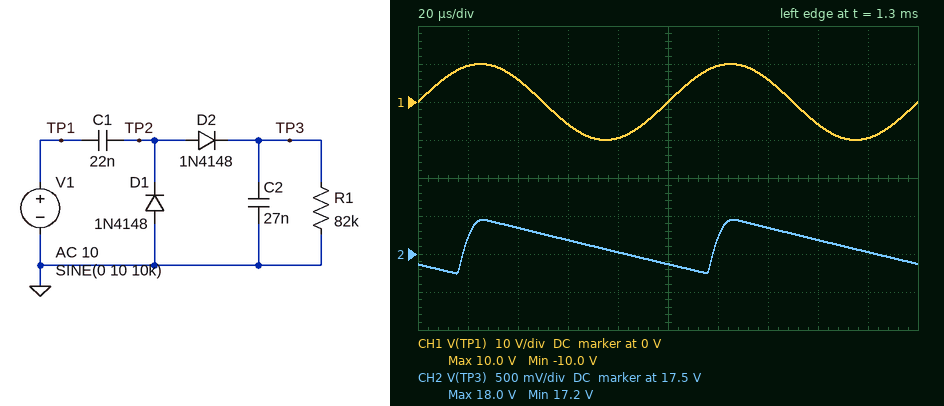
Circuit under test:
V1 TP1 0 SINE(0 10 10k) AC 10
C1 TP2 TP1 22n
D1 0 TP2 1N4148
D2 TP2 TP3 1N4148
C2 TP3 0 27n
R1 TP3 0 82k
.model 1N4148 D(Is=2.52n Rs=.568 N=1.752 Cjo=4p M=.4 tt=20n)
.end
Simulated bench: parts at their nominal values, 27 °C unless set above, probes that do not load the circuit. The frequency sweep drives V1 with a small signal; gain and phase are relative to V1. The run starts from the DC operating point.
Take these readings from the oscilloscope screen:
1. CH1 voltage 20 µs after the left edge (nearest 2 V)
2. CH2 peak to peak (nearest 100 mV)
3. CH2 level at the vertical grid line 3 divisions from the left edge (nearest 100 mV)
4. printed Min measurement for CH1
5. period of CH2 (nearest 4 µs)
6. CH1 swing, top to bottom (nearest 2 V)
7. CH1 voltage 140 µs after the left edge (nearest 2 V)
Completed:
10 V
700 mV
17.7 V
-10.0 V
100 µs
20 V
6 V
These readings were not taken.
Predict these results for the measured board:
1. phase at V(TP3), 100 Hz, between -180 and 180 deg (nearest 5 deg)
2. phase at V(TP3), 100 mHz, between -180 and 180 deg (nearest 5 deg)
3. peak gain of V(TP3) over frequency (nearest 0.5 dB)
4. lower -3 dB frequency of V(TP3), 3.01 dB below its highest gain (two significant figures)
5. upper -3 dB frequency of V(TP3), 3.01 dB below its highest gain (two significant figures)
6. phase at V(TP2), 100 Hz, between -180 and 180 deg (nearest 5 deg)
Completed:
-50 deg
85 deg
-47.0 dB
790 mHz
74 Hz
0 deg
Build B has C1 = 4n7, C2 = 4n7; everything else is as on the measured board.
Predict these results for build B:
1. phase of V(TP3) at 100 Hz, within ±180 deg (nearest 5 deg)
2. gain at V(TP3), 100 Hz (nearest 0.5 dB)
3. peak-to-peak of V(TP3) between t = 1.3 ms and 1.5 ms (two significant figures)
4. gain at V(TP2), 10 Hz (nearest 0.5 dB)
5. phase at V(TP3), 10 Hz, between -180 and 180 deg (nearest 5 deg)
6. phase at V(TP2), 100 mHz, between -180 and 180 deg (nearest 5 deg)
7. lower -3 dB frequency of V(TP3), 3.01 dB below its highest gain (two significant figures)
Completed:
-10 deg
-47.0 dB
2.9 V
-0.5 dB
20 deg
90 deg
3.7 Hz
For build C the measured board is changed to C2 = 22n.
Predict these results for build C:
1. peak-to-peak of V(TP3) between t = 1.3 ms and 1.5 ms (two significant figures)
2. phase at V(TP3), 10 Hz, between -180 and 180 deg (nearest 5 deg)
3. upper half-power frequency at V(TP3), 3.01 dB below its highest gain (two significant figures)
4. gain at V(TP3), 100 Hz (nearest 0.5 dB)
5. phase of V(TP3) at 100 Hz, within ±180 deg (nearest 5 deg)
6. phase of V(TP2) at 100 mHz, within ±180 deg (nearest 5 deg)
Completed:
860 mV
0 deg
90 Hz
-50.5 dB
-45 deg
85 deg
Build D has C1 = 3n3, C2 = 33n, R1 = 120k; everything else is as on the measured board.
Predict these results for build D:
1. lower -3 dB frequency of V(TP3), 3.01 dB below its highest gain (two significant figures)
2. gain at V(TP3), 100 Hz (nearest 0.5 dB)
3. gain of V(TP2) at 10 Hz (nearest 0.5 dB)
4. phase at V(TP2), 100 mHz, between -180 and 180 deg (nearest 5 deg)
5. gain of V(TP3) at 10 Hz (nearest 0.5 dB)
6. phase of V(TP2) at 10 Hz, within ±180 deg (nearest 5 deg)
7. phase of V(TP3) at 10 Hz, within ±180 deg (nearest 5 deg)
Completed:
4.3 Hz
-52.0 dB
-1.0 dB
90 deg
-45.0 dB
30 deg
15 deg
